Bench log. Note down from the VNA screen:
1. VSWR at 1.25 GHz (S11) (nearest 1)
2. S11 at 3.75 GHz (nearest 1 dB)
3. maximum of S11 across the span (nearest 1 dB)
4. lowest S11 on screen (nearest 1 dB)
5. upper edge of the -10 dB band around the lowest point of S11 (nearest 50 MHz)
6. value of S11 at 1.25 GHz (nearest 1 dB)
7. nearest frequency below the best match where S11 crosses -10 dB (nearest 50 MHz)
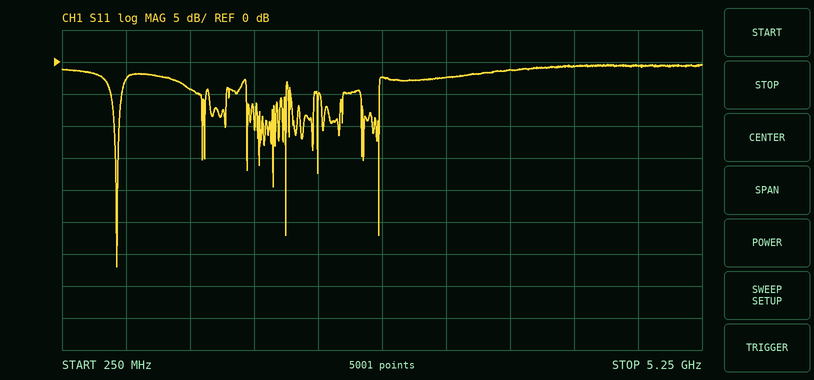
4
-1 dB
0 dB
-32 dB
700 MHz
-4 dB
650 MHz
